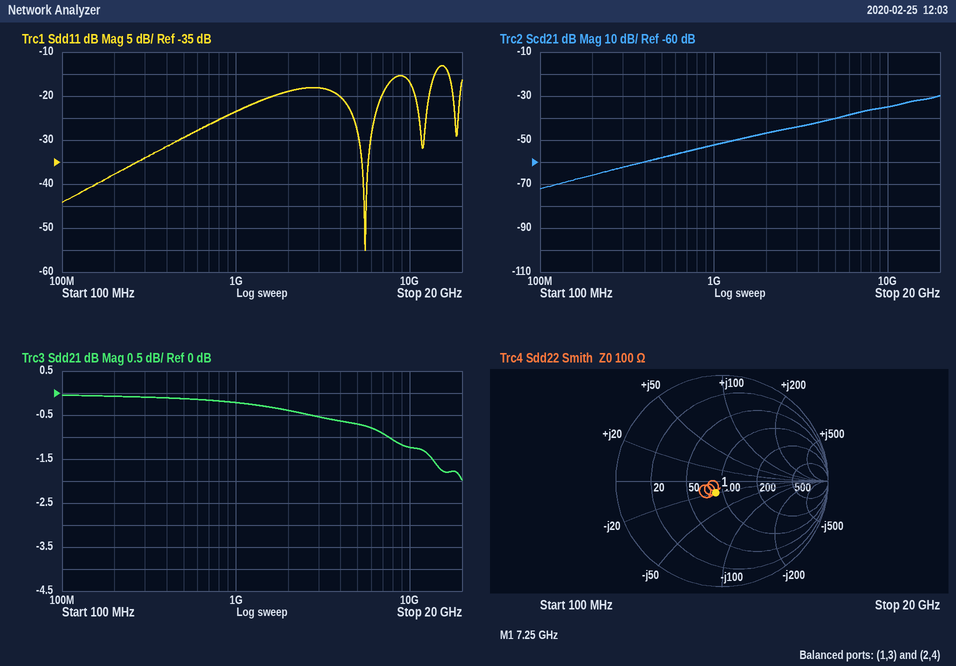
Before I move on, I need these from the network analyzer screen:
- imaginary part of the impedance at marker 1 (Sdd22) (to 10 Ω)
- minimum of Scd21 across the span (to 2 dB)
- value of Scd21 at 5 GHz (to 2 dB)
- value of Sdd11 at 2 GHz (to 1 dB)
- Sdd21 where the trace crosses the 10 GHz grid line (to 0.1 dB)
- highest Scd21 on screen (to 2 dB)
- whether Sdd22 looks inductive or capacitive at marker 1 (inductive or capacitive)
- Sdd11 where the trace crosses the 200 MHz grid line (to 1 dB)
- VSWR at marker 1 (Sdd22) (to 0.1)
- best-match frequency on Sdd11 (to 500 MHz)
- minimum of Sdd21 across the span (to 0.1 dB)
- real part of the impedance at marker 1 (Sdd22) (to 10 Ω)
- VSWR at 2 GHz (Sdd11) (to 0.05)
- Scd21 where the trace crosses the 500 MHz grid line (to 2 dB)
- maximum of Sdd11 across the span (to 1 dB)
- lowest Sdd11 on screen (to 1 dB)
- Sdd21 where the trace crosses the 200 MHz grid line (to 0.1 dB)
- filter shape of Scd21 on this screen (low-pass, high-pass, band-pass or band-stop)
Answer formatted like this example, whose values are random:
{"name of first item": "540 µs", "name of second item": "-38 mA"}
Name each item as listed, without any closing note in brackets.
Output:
{"imaginary part of the impedance at marker 1 (Sdd22)": "-20 Ω", "minimum of Scd21 across the span": "-72 dB", "value of Scd21 at 5 GHz": "-40 dB", "value of Sdd11 at 2 GHz": "-19 dB", "Sdd21 where the trace crosses the 10 GHz grid line": "-1.2 dB", "highest Scd21 on screen": "-30 dB", "whether Sdd22 looks inductive or capacitive at marker 1": "capacitive", "Sdd11 where the trace crosses the 200 MHz grid line": "-38 dB", "VSWR at marker 1 (Sdd22)": "1.3", "best-match frequency on Sdd11": "5.5 GHz", "minimum of Sdd21 across the span": "-2.0 dB", "real part of the impedance at marker 1 (Sdd22)": "90 Ω", "VSWR at 2 GHz (Sdd11)": "1.25", "Scd21 where the trace crosses the 500 MHz grid line": "-58 dB", "maximum of Sdd11 across the span": "-13 dB", "lowest Sdd11 on screen": "-55 dB", "Sdd21 where the trace crosses the 200 MHz grid line": "-0.1 dB", "filter shape of Scd21 on this screen": "high-pass"}
